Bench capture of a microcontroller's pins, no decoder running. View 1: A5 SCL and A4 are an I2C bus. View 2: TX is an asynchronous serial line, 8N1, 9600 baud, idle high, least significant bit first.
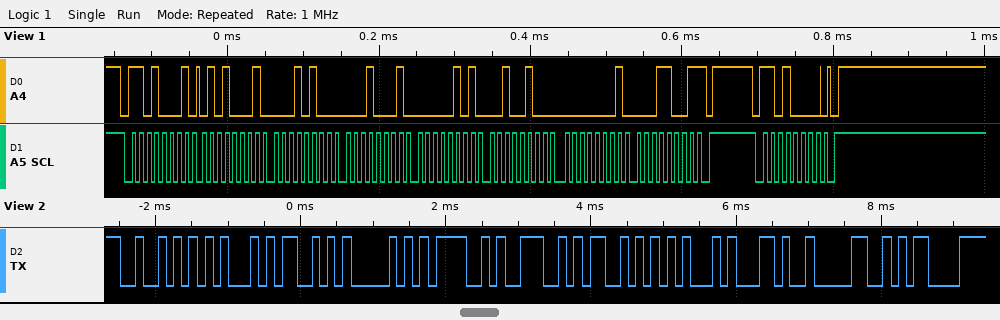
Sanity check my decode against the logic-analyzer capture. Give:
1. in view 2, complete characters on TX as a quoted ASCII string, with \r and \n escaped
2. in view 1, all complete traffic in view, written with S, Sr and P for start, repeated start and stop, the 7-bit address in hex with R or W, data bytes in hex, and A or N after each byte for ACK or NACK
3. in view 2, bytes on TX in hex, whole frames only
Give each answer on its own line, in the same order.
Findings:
"RESPONSE,0\r"
S 68R A 51 A 14 A 11 A 05 A 24 A 01 A 19 N P S 68W A P
52 45 53 50 4F 4E 53 45 2C 30 0D
